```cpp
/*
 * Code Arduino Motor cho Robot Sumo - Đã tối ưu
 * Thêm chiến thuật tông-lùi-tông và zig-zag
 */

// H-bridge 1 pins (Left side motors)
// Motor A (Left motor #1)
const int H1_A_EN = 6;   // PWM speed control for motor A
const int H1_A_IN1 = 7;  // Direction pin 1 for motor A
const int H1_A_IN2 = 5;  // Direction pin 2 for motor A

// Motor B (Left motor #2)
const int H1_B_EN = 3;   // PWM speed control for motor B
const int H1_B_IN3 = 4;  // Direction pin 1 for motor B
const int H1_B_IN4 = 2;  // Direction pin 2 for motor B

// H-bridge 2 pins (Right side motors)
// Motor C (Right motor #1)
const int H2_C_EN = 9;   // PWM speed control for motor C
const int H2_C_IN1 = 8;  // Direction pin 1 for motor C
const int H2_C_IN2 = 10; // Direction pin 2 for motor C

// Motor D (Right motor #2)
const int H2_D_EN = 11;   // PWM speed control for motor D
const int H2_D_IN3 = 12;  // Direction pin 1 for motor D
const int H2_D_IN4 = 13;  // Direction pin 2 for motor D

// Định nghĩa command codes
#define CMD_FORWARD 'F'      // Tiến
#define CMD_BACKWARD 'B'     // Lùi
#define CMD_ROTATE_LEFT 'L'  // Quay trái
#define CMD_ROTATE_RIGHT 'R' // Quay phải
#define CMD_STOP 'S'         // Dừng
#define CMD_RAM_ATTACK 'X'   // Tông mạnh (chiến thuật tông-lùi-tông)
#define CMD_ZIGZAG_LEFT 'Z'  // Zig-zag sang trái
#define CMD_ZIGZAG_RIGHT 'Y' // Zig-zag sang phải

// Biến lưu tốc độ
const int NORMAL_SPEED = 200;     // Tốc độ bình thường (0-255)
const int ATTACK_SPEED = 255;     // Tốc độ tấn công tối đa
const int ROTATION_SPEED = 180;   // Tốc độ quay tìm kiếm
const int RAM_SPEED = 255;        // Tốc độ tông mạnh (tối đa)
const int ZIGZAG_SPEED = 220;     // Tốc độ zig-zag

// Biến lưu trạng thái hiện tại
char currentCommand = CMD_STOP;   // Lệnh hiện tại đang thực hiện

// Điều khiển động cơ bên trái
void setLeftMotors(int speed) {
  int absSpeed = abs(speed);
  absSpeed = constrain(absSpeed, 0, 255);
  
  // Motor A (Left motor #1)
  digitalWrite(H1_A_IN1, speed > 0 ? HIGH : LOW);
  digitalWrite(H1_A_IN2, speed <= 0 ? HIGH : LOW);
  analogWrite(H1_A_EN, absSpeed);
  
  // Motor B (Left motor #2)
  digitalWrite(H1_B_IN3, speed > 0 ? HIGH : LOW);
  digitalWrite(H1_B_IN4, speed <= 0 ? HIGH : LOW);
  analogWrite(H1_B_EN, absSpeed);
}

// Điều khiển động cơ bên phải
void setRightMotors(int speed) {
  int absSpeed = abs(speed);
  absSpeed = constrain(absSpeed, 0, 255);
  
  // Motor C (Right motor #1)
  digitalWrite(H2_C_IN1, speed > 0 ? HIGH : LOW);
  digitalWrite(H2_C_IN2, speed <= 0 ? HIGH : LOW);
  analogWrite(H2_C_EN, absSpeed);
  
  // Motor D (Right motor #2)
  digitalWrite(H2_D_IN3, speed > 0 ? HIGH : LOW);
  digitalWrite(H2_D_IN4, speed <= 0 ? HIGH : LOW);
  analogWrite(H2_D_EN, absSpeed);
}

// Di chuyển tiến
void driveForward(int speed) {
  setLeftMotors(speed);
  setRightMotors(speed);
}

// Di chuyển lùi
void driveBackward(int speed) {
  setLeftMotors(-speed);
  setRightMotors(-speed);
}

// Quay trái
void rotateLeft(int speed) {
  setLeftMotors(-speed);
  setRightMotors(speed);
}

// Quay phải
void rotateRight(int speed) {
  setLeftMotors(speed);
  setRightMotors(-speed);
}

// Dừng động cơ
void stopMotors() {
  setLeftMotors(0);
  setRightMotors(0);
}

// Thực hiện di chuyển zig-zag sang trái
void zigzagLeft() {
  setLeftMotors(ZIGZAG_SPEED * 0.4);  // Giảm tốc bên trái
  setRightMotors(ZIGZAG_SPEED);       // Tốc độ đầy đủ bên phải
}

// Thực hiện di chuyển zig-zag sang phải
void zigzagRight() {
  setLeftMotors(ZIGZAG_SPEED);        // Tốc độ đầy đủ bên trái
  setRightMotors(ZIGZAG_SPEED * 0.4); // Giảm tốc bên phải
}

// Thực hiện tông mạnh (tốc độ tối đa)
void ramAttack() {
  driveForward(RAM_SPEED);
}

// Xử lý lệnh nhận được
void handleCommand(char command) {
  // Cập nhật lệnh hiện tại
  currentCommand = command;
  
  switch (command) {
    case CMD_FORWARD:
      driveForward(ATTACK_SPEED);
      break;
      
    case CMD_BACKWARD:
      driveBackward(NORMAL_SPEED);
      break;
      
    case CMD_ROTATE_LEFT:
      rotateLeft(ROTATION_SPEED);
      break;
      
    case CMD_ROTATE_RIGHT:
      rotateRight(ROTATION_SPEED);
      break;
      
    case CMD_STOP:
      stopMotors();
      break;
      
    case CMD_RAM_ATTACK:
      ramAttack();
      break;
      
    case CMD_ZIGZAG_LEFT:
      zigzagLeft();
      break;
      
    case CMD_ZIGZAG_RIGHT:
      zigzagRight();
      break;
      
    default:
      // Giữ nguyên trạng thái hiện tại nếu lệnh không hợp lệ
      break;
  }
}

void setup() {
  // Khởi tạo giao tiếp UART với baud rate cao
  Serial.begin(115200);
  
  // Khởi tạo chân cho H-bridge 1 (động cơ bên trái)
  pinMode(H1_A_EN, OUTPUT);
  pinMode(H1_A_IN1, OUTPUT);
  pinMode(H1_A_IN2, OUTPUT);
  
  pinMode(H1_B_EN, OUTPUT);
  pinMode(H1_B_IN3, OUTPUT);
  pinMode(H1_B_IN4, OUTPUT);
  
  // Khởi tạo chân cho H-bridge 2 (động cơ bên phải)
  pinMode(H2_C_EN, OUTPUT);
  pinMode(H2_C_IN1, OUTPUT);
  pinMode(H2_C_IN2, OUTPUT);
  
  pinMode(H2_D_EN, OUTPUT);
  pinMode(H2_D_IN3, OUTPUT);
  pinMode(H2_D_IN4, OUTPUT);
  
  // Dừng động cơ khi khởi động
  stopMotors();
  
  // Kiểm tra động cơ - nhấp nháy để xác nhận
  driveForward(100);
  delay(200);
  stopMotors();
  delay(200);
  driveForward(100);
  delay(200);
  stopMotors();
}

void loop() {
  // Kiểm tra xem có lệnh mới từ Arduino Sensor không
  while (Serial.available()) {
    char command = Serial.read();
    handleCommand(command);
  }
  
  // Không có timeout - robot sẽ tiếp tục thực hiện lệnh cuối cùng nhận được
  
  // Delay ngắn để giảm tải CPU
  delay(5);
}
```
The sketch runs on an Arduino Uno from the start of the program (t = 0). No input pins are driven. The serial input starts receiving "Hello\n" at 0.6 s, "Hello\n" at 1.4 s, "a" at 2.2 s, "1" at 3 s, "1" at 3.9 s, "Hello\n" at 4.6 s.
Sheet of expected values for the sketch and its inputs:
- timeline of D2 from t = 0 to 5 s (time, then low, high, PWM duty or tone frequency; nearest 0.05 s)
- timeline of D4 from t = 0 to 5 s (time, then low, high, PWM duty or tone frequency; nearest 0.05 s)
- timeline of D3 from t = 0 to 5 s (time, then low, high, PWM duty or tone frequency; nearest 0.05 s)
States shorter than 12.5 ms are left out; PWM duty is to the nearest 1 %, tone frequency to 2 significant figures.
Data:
0 s low; 0.2 s high; 0.4 s low; 0.6 s high
0 s high; 0.2 s low; 0.4 s high; 0.6 s low
0 s PWM 39 %; 0.2 s low; 0.4 s PWM 39 %; 0.6 s low
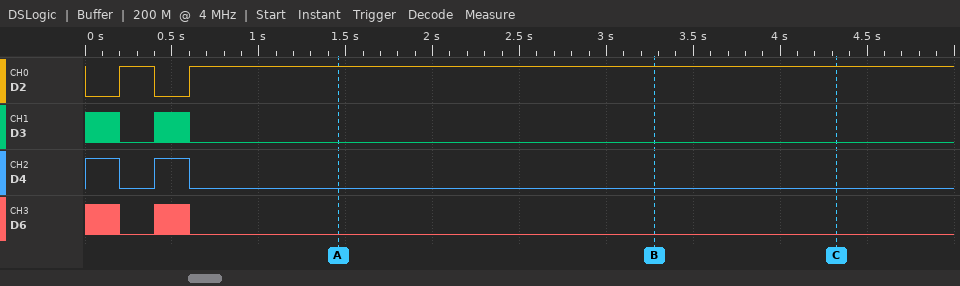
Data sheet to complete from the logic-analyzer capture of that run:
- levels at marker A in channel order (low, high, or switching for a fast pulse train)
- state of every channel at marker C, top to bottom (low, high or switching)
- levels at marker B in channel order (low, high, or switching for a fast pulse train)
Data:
D2 high, D3 low, D4 low, D6 low
D2 high, D3 low, D4 low, D6 low
D2 high, D3 low, D4 low, D6 low
